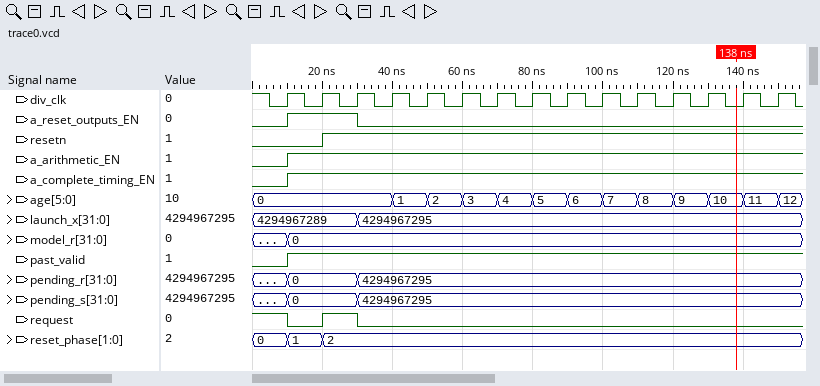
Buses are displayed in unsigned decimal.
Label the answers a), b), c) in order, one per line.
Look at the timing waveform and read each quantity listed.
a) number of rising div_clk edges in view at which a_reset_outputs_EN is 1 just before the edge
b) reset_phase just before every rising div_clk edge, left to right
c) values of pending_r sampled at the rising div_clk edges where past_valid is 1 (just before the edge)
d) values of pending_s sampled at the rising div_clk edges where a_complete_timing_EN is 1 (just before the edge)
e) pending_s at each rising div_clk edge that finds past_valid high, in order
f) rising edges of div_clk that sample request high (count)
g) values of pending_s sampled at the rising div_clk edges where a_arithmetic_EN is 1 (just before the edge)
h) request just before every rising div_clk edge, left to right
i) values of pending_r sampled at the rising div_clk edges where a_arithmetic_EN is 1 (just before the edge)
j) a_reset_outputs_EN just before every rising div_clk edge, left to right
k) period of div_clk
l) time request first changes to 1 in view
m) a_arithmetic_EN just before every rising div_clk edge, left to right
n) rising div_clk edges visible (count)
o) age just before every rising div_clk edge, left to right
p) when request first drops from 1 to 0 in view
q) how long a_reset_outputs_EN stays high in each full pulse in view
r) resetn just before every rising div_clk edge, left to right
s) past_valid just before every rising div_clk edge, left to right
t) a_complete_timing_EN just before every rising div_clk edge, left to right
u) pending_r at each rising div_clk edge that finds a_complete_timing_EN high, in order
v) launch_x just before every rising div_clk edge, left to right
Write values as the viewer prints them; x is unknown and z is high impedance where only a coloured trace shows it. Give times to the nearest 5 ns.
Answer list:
a) 2
b) 0, 1, 2, 2, 2, 2, 2, 2, 2, 2, 2, 2, 2, 2, 2
c) 0, 0, 4294967295, 4294967295, 4294967295, 4294967295, 4294967295, 4294967295, 4294967295, 4294967295, 4294967295, 4294967295, 4294967295, 4294967295
d) 0, 0, 4294967295, 4294967295, 4294967295, 4294967295, 4294967295, 4294967295, 4294967295, 4294967295, 4294967295, 4294967295, 4294967295, 4294967295
e) 0, 0, 4294967295, 4294967295, 4294967295, 4294967295, 4294967295, 4294967295, 4294967295, 4294967295, 4294967295, 4294967295, 4294967295, 4294967295
f) 2
g) 0, 0, 4294967295, 4294967295, 4294967295, 4294967295, 4294967295, 4294967295, 4294967295, 4294967295, 4294967295, 4294967295, 4294967295, 4294967295
h) 1 0 1 0 0 0 0 0 0 0 0 0 0 0 0
i) 0, 0, 4294967295, 4294967295, 4294967295, 4294967295, 4294967295, 4294967295, 4294967295, 4294967295, 4294967295, 4294967295, 4294967295, 4294967295
j) 0 1 1 0 0 0 0 0 0 0 0 0 0 0 0
k) 10 ns
l) 20 ns
m) 0 1 1 1 1 1 1 1 1 1 1 1 1 1 1
n) 15
o) 0, 0, 0, 0, 1, 2, 3, 4, 5, 6, 7, 8, 9, 10, 11
p) 10 ns
q) 20 ns
r) 0 0 1 1 1 1 1 1 1 1 1 1 1 1 1
s) 0 1 1 1 1 1 1 1 1 1 1 1 1 1 1
t) 0 1 1 1 1 1 1 1 1 1 1 1 1 1 1
u) 0, 0, 4294967295, 4294967295, 4294967295, 4294967295, 4294967295, 4294967295, 4294967295, 4294967295, 4294967295, 4294967295, 4294967295, 4294967295
v) 4294967289, 4294967289, 4294967289, 4294967295, 4294967295, 4294967295, 4294967295, 4294967295, 4294967295, 4294967295, 4294967295, 4294967295, 4294967295, 4294967295, 4294967295
